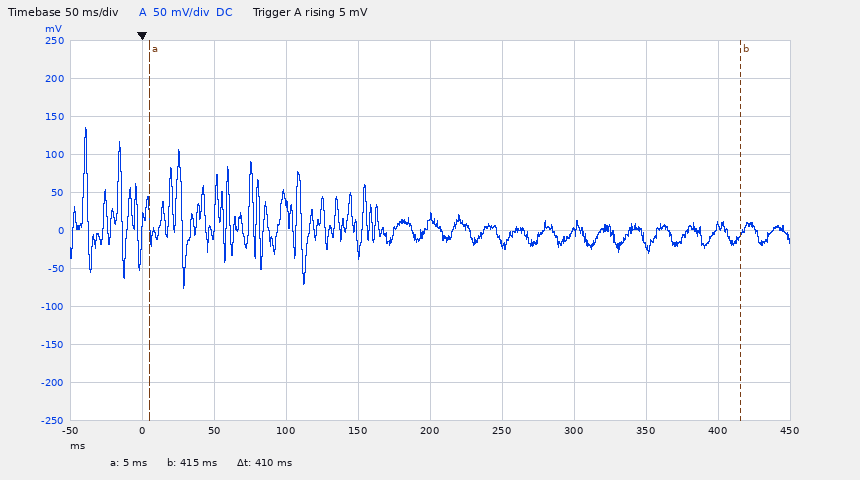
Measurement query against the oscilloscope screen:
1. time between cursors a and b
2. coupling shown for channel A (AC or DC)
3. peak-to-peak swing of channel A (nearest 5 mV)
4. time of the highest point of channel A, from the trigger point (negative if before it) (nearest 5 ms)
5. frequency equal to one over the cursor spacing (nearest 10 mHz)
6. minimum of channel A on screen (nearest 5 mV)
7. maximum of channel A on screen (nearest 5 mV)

410 ms
DC
210 mV
-40 ms
2.44 Hz
-75 mV
135 mV
